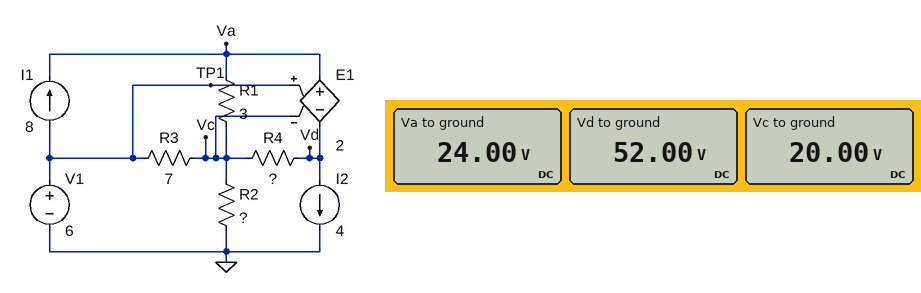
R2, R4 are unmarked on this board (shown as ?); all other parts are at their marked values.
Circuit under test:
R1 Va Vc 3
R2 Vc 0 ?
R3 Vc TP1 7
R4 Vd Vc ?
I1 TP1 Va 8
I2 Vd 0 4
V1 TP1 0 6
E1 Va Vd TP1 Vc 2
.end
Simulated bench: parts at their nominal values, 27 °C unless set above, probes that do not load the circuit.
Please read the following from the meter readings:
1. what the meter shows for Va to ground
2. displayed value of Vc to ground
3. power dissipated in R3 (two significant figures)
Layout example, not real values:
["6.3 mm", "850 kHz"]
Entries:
["24.00 V", "20.00 V", "28 W"]
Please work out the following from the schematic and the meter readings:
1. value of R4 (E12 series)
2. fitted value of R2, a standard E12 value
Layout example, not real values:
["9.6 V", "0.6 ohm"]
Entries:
["12 Ω", "10 Ω"]
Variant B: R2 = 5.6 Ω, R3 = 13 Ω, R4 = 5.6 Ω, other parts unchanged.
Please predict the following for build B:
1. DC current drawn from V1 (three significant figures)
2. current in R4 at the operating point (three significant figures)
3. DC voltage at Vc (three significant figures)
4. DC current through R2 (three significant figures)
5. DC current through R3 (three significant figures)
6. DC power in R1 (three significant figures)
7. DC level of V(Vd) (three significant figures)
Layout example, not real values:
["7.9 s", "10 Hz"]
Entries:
["7.12 A", "4.06 A", "17.5 V", "3.12 A", "882 mA", "11.2 mW", "40.2 V"]
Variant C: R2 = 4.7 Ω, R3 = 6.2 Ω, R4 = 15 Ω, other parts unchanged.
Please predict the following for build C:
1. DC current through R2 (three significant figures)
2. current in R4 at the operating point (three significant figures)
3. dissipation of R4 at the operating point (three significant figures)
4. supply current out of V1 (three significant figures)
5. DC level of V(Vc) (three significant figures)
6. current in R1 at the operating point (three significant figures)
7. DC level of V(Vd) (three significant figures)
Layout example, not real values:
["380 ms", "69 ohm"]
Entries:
["2.83 A", "1.48 A", "32.7 W", "6.83 A", "13.3 V", "2.52 A", "35.4 V"]
